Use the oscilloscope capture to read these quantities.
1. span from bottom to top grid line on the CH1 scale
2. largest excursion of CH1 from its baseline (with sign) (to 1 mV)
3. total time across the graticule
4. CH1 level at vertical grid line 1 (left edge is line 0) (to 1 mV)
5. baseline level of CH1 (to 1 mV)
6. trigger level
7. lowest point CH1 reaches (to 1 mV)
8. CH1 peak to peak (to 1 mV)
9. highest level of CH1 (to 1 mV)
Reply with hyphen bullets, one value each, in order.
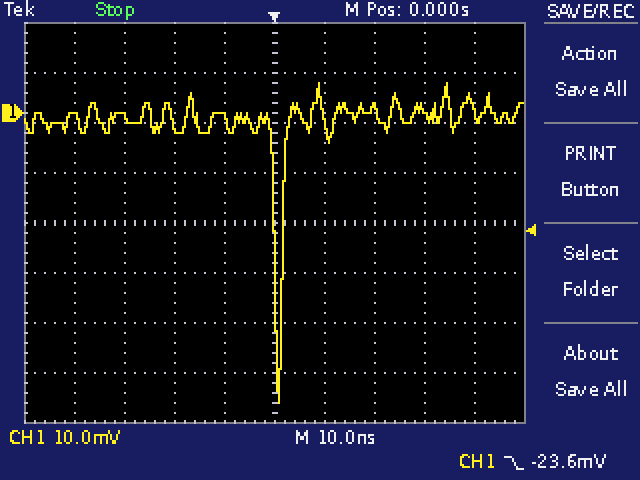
- 80 mV
- -57 mV
- 100 ns
- -1 mV
- -1 mV
- -23.6 mV
- -58 mV
- 64 mV
- 6 mV
